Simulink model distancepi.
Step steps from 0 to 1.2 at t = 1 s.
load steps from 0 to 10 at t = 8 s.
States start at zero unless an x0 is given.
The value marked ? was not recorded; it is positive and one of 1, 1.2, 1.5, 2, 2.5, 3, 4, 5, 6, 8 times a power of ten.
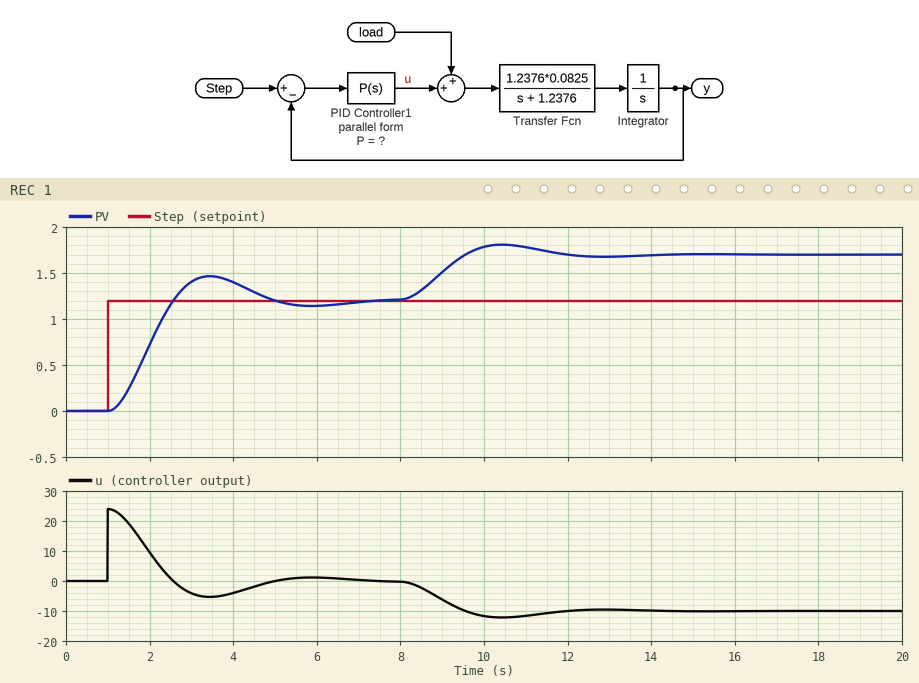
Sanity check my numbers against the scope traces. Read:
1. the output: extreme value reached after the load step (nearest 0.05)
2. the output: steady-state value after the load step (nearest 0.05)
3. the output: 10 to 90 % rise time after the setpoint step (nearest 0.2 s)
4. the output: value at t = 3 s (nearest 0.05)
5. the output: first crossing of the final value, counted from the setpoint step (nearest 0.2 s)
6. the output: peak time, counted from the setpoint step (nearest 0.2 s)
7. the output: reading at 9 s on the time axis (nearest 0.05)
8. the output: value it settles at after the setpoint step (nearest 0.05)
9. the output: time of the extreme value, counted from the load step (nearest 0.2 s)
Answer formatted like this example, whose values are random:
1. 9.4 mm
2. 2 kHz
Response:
1. 1.80
2. 1.70
3. 1.0 s
4. 1.40
5. 1.6 s
6. 2.4 s
7. 1.50
8. 1.20
9. 2.4 s
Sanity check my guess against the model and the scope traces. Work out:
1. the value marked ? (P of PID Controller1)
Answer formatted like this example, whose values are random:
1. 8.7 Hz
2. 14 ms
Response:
1. 20
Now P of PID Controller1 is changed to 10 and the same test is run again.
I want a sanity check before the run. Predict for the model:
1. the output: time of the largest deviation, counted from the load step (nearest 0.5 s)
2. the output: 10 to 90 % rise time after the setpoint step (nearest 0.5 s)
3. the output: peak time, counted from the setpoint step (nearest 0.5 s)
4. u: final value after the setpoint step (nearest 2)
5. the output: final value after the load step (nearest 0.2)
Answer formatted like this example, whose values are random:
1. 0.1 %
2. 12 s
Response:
1. 4.0 s
2. 2.0 s
3. 4.0 s
4. 0
5. 2.2
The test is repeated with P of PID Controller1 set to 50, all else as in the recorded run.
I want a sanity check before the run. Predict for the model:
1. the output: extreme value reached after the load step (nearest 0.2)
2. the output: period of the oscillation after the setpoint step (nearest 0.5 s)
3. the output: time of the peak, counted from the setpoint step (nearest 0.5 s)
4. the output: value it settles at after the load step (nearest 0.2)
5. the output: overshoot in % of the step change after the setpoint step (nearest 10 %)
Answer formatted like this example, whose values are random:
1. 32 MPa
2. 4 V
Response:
1. 1.4
2. 3.0 s
3. 1.5 s
4. 1.4
5. 40 %
